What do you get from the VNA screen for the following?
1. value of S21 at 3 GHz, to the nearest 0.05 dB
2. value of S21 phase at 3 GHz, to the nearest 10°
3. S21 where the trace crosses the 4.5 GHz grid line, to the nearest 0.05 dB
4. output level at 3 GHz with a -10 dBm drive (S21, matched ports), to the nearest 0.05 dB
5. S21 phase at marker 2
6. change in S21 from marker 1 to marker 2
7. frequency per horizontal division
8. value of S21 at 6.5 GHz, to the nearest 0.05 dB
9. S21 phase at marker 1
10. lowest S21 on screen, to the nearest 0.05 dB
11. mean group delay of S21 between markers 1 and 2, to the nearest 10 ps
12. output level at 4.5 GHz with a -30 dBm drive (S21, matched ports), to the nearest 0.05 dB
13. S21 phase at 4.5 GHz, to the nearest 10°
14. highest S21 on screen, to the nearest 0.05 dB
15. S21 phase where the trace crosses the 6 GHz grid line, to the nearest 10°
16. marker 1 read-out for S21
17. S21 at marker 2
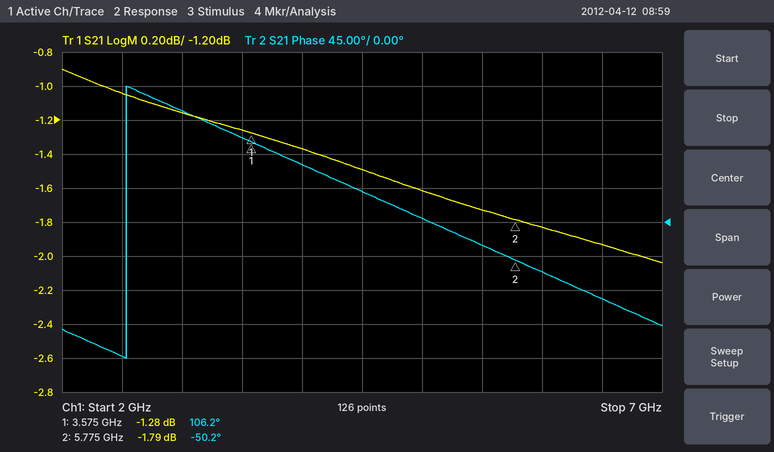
-1.15 dB
150°
-1.50 dB
-11.15 dBm
-50.2°
-0.51 dB
500 MHz
-1.95 dB
106.2°
-2.05 dB
200 ps
-31.50 dBm
40°
-0.90 dB
-70°
-1.28 dB
-1.79 dB
